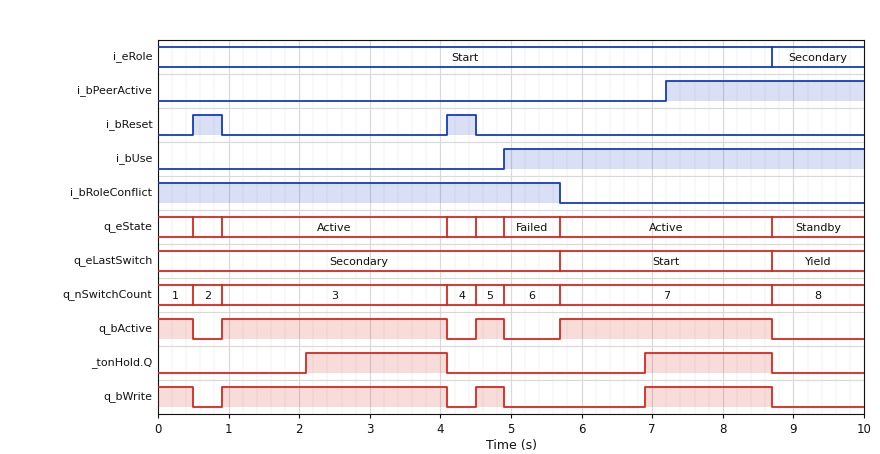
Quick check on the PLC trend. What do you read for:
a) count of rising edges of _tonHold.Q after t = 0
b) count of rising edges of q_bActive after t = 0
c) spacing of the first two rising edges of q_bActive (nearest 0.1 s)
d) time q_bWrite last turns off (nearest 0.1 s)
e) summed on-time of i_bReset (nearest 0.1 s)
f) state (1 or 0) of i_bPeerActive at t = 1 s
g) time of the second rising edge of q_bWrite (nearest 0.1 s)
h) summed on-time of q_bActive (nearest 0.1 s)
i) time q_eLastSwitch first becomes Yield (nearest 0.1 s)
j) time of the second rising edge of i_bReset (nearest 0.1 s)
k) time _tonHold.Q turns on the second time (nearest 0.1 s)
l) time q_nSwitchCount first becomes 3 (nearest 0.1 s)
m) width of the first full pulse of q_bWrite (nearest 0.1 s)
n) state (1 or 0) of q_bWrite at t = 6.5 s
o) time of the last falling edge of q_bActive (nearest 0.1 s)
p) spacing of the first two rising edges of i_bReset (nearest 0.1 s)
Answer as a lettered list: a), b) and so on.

a) 2
b) 3
c) 3.6 s
d) 8.7 s
e) 0.8 s
f) 0
g) 4.5 s
h) 7.1 s
i) 8.7 s
j) 4.1 s
k) 6.9 s
l) 0.9 s
m) 3.2 s
n) 0
o) 8.7 s
p) 3.6 s
